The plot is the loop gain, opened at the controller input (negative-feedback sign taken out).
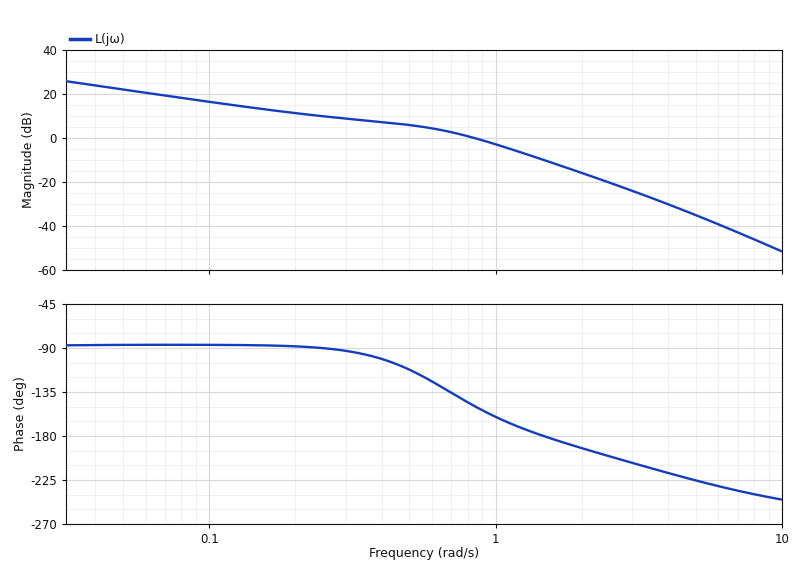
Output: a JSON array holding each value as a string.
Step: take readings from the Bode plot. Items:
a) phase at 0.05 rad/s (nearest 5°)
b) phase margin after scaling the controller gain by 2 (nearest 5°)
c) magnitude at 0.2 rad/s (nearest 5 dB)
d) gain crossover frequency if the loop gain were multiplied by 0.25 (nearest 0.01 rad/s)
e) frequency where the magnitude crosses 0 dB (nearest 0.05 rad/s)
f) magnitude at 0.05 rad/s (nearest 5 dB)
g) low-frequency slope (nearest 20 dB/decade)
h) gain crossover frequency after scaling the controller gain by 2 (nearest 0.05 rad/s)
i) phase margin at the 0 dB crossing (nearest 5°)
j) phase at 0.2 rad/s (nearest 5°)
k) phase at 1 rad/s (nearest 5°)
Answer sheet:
["-85°", "10°", "10 dB", "0.18 rad/s", "0.85 rad/s", "20 dB", "-20 dB/decade", "1.20 rad/s", "30°", "-90°", "-160°"]
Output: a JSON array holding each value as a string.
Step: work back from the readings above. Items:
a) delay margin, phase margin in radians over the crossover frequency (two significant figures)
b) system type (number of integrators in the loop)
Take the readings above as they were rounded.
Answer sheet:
["0.62 s", "1"]
